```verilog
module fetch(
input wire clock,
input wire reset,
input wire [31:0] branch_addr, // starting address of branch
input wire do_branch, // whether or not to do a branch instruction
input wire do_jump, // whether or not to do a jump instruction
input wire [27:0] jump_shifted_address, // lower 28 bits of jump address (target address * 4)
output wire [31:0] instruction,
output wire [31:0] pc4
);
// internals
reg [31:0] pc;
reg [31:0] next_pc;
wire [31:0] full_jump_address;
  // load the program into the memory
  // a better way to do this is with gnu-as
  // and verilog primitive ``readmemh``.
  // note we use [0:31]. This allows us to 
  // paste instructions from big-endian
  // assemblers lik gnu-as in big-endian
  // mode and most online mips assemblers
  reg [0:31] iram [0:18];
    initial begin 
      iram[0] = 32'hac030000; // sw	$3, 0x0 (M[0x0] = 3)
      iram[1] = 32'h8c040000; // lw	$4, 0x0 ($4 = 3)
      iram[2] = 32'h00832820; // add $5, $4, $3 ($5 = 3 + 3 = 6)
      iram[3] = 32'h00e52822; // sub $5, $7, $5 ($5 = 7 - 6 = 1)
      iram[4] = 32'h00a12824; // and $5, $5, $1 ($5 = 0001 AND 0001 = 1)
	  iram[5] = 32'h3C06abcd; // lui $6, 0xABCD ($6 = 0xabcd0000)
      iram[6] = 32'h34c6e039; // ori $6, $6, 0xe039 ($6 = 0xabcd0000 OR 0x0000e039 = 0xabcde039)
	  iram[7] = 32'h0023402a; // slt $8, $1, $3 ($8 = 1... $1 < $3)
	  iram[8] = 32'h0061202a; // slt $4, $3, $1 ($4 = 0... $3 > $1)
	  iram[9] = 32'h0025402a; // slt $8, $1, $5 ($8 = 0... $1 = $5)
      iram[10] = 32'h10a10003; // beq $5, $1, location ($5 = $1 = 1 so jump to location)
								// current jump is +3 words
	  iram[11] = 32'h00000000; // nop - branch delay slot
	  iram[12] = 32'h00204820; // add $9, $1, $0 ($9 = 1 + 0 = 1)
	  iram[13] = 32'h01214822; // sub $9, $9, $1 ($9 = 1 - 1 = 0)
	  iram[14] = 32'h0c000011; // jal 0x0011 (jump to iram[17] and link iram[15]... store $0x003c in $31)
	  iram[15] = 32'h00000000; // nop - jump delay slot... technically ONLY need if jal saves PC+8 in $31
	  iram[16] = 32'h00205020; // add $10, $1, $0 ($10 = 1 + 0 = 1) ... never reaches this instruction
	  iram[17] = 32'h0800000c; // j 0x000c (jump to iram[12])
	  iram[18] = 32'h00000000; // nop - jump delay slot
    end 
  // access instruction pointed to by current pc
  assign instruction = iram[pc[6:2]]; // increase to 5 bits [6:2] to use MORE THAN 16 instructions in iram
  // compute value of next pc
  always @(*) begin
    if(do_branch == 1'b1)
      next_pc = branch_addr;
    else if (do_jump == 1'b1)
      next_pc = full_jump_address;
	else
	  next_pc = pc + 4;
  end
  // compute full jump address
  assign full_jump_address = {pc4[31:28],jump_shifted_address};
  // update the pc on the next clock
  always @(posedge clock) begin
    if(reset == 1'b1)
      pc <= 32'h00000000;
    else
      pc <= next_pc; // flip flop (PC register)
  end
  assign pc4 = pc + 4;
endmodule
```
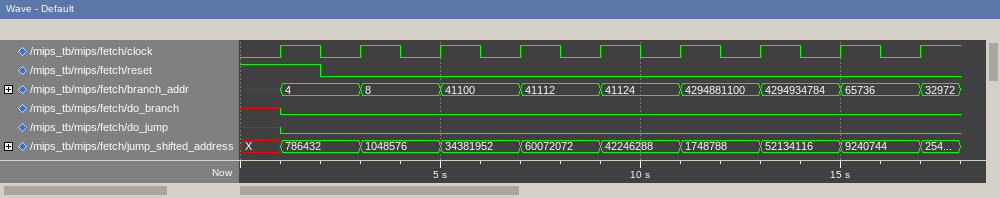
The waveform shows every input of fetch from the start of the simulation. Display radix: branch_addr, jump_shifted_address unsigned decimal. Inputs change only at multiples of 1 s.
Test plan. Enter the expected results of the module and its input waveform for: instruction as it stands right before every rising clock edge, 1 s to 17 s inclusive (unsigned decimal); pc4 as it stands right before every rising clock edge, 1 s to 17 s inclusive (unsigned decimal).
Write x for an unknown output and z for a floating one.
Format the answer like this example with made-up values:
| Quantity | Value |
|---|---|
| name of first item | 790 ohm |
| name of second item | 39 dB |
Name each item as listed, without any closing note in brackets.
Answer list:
| Quantity | Value |
|---|---|
| instruction as it stands right before every rising clock edge, 1 s to 17 s inclusive | x, 2885877760, 2349072384, 8595488, 15018018, 10561572, 1007070157, 885448761, 2310186 |
| pc4 as it stands right before every rising clock edge, 1 s to 17 s inclusive | x, 4, 8, 12, 16, 20, 24, 28, 32 |
